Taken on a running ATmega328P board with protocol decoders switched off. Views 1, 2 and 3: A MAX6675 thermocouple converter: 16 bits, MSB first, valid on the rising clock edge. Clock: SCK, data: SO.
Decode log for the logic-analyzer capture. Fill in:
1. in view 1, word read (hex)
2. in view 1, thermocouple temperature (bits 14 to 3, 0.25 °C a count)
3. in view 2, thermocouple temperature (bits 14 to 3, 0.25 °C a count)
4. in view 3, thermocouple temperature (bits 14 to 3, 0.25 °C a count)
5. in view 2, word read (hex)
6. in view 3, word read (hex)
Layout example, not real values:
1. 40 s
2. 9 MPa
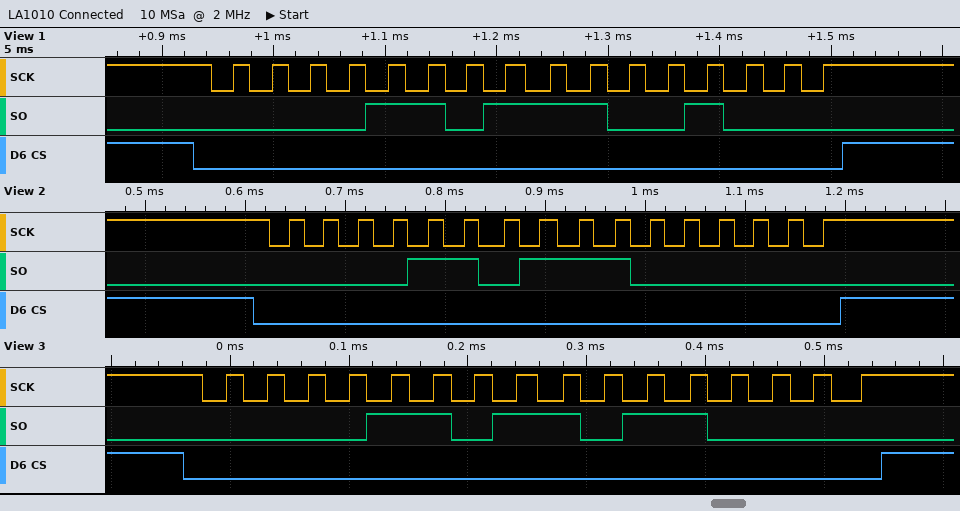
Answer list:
1. 0x0DC8
2. 110.25 °C
3. 110.00 °C
4. 109.50 °C
5. 0x0DC0
6. 0x0DB0
